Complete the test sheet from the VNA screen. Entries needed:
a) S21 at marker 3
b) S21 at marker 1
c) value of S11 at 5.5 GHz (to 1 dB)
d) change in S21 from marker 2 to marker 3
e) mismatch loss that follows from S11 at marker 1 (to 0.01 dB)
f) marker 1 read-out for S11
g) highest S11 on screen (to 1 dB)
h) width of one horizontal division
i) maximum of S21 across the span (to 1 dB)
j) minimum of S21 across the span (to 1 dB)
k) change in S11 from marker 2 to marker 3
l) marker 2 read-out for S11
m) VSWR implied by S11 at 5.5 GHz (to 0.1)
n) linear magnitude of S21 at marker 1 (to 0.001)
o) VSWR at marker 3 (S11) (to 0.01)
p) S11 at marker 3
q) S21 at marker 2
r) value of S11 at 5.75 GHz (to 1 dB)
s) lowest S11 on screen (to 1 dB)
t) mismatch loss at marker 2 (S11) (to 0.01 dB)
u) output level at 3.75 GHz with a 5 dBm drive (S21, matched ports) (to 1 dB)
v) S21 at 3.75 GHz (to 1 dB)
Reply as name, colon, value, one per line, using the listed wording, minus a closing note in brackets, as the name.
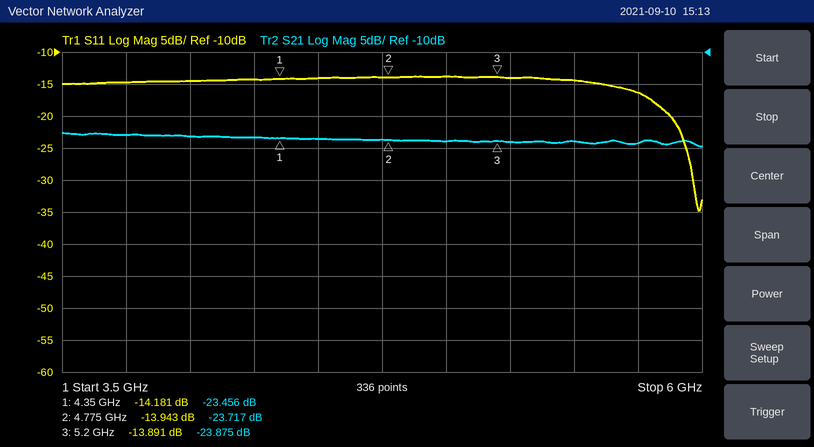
S21 at marker 3: -23.875 dB
S21 at marker 1: -23.456 dB
value of S11 at 5.5 GHz: -14 dB
change in S21 from marker 2 to marker 3: -0.158 dB
mismatch loss that follows from S11 at marker 1: 0.17 dB
marker 1 read-out for S11: -14.181 dB
highest S11 on screen: -14 dB
width of one horizontal division: 250 MHz
maximum of S21 across the span: -23 dB
minimum of S21 across the span: -25 dB
change in S11 from marker 2 to marker 3: 0.052 dB
marker 2 read-out for S11: -13.943 dB
VSWR implied by S11 at 5.5 GHz: 1.5
linear magnitude of S21 at marker 1: 0.067
VSWR at marker 3 (S11): 1.51
S11 at marker 3: -13.891 dB
S21 at marker 2: -23.717 dB
value of S11 at 5.75 GHz: -16 dB
lowest S11 on screen: -35 dB
mismatch loss at marker 2 (S11): 0.18 dB
output level at 3.75 GHz with a 5 dBm drive (S21, matched ports): -18 dBm
S21 at 3.75 GHz: -23 dB
